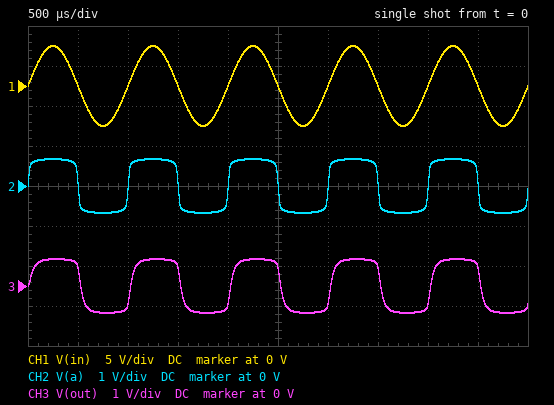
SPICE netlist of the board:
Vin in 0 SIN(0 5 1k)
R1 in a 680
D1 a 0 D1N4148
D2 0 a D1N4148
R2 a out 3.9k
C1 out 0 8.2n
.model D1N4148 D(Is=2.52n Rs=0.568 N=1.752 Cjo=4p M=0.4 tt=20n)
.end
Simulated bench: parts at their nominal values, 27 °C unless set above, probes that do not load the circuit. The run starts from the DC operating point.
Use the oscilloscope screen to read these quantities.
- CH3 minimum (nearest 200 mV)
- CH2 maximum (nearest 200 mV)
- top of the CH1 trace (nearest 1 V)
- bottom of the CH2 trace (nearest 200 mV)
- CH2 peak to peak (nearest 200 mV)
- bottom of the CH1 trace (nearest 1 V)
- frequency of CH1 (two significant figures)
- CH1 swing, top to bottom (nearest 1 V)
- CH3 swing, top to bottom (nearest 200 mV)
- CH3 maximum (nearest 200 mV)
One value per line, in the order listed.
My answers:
-600 mV
600 mV
5 V
-600 mV
1.4 V
-5 V
1.0 kHz
10 V
1.4 V
600 mV
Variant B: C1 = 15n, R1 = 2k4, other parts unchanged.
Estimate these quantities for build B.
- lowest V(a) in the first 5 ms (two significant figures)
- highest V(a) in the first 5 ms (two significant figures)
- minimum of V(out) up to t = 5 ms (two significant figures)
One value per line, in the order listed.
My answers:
-610 mV
610 mV
-600 mV
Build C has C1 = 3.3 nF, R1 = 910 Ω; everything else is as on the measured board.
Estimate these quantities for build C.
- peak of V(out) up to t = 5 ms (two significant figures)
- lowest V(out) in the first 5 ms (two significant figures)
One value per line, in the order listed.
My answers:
660 mV
-660 mV
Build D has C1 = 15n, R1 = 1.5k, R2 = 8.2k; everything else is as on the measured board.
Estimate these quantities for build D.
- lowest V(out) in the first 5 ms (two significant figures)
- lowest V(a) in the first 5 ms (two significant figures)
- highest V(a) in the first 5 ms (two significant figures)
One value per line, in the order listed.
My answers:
-580 mV
-630 mV
630 mV
